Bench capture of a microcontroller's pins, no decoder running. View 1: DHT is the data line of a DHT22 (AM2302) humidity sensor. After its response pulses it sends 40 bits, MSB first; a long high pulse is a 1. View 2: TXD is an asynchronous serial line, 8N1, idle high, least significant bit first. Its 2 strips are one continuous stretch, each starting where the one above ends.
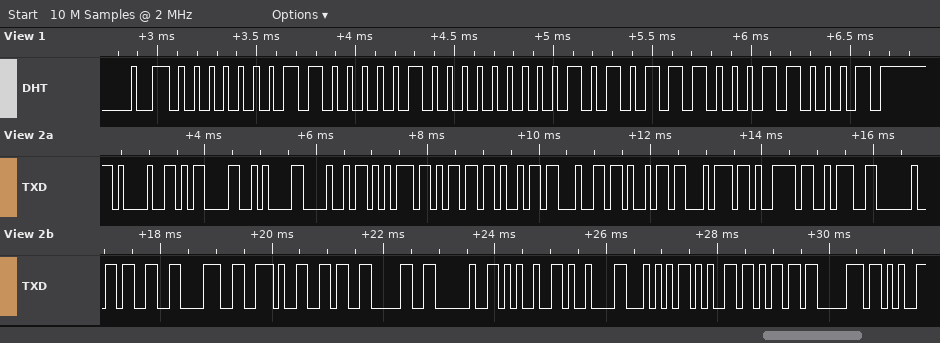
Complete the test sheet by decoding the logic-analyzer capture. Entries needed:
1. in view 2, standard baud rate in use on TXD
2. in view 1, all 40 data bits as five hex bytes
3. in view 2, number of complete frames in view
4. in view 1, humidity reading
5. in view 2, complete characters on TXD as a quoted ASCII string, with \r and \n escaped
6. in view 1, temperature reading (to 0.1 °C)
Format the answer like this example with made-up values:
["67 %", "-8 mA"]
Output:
["9600 baud", "01 82 00 AE 31", "25", "38.6 %", "\"!\\r\\nHumidity: 38.60 %\\tTemp\"", "17.4 °C"]
